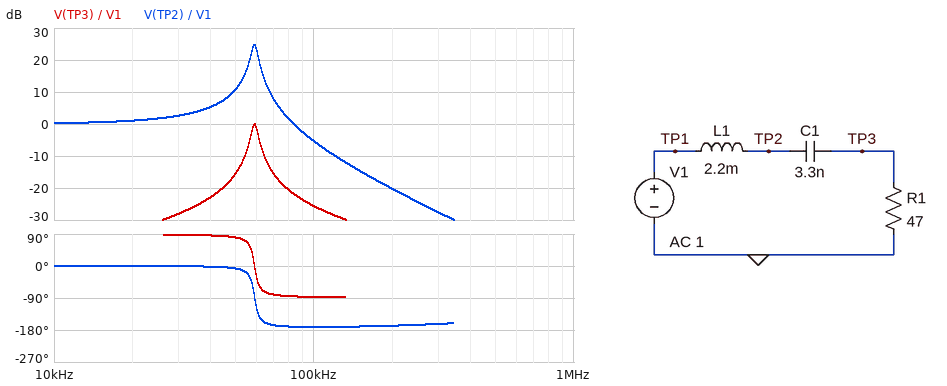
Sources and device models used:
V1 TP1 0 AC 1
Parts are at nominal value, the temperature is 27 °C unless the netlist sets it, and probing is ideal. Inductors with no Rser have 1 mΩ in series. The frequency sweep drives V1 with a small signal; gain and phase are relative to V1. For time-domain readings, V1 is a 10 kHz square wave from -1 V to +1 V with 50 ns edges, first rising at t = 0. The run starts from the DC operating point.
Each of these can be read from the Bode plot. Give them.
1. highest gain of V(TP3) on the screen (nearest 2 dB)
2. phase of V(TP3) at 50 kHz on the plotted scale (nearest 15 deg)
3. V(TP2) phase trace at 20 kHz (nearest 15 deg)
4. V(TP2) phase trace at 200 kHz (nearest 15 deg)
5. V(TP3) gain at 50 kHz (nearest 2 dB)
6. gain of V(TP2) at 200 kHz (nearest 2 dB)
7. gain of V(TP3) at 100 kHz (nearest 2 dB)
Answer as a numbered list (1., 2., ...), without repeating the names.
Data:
1. 0 dB
2. 75 deg
3. 0 deg
4. -165 deg
5. -16 dB
6. -20 dB
7. -26 dB
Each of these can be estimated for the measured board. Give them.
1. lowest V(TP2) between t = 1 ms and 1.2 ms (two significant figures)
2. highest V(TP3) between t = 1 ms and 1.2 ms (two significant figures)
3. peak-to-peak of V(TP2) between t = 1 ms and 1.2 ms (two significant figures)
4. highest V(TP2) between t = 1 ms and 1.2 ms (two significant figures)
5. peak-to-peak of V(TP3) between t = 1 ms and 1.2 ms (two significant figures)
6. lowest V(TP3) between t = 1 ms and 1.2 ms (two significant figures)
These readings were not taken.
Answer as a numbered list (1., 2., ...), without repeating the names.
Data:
1. -2.2 V
2. 70 mV
3. 4.3 V
4. 2.2 V
5. 140 mV
6. -70 mV
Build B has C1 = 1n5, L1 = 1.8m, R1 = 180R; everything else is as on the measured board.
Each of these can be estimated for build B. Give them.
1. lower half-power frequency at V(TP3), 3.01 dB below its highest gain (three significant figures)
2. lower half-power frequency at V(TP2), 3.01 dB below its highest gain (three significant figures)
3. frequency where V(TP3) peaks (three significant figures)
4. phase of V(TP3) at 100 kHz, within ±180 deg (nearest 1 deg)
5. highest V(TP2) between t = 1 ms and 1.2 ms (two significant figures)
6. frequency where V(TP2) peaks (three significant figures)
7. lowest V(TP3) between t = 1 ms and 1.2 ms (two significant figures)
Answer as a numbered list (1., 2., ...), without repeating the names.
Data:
1. 89.2 kHz
2. 87.9 kHz
3. 96.9 kHz
4. -21 deg
5. 2.5 V
6. 96.2 kHz
7. -280 mV
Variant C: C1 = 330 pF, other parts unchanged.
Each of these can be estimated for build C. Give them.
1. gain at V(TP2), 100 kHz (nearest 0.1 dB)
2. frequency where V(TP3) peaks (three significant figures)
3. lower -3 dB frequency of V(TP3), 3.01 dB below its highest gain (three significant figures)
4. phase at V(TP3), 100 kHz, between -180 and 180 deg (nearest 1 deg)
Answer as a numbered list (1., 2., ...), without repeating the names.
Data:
1. 2.9 dB
2. 187 kHz
3. 185 kHz
4. 89 deg
